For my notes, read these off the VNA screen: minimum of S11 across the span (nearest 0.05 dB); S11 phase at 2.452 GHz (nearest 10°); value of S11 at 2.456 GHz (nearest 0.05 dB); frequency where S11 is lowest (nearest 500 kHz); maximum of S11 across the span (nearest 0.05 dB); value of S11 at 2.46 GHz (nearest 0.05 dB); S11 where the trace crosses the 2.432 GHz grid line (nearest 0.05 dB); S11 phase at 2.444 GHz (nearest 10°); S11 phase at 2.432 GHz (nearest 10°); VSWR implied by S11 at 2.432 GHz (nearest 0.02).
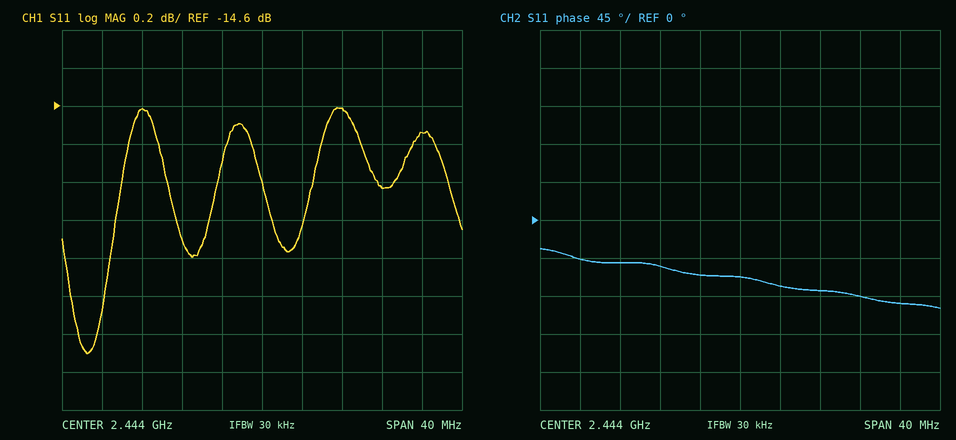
-15.90 dB
-80°
-15.05 dB
2.4265 GHz
-14.60 dB
-14.75 dB
-14.60 dB
-70°
-50°
1.46
